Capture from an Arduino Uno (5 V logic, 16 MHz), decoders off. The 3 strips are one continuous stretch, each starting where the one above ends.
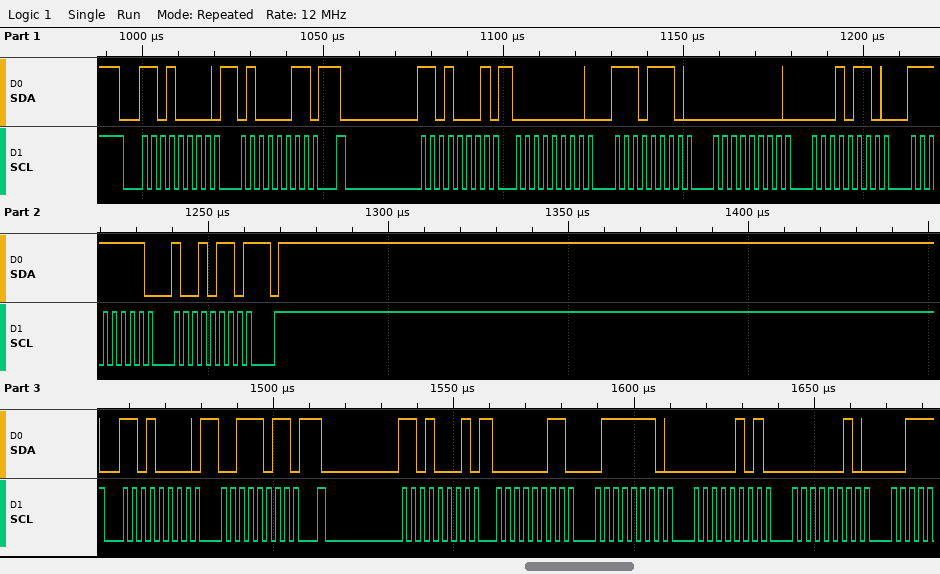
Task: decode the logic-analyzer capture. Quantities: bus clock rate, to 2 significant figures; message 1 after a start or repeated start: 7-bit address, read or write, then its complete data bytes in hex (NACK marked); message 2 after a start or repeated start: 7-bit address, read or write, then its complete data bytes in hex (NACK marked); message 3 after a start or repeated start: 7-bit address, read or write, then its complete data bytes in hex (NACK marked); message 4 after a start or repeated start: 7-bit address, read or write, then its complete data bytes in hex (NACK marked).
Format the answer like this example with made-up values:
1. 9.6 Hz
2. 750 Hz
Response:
1. 400 kHz
2. 0x68 write: 43
3. 0x68 read: 00 EE 00 16 FF 96 NACK
4. 0x68 write: 3B
5. 0x68 read: 03 7E 05 02
